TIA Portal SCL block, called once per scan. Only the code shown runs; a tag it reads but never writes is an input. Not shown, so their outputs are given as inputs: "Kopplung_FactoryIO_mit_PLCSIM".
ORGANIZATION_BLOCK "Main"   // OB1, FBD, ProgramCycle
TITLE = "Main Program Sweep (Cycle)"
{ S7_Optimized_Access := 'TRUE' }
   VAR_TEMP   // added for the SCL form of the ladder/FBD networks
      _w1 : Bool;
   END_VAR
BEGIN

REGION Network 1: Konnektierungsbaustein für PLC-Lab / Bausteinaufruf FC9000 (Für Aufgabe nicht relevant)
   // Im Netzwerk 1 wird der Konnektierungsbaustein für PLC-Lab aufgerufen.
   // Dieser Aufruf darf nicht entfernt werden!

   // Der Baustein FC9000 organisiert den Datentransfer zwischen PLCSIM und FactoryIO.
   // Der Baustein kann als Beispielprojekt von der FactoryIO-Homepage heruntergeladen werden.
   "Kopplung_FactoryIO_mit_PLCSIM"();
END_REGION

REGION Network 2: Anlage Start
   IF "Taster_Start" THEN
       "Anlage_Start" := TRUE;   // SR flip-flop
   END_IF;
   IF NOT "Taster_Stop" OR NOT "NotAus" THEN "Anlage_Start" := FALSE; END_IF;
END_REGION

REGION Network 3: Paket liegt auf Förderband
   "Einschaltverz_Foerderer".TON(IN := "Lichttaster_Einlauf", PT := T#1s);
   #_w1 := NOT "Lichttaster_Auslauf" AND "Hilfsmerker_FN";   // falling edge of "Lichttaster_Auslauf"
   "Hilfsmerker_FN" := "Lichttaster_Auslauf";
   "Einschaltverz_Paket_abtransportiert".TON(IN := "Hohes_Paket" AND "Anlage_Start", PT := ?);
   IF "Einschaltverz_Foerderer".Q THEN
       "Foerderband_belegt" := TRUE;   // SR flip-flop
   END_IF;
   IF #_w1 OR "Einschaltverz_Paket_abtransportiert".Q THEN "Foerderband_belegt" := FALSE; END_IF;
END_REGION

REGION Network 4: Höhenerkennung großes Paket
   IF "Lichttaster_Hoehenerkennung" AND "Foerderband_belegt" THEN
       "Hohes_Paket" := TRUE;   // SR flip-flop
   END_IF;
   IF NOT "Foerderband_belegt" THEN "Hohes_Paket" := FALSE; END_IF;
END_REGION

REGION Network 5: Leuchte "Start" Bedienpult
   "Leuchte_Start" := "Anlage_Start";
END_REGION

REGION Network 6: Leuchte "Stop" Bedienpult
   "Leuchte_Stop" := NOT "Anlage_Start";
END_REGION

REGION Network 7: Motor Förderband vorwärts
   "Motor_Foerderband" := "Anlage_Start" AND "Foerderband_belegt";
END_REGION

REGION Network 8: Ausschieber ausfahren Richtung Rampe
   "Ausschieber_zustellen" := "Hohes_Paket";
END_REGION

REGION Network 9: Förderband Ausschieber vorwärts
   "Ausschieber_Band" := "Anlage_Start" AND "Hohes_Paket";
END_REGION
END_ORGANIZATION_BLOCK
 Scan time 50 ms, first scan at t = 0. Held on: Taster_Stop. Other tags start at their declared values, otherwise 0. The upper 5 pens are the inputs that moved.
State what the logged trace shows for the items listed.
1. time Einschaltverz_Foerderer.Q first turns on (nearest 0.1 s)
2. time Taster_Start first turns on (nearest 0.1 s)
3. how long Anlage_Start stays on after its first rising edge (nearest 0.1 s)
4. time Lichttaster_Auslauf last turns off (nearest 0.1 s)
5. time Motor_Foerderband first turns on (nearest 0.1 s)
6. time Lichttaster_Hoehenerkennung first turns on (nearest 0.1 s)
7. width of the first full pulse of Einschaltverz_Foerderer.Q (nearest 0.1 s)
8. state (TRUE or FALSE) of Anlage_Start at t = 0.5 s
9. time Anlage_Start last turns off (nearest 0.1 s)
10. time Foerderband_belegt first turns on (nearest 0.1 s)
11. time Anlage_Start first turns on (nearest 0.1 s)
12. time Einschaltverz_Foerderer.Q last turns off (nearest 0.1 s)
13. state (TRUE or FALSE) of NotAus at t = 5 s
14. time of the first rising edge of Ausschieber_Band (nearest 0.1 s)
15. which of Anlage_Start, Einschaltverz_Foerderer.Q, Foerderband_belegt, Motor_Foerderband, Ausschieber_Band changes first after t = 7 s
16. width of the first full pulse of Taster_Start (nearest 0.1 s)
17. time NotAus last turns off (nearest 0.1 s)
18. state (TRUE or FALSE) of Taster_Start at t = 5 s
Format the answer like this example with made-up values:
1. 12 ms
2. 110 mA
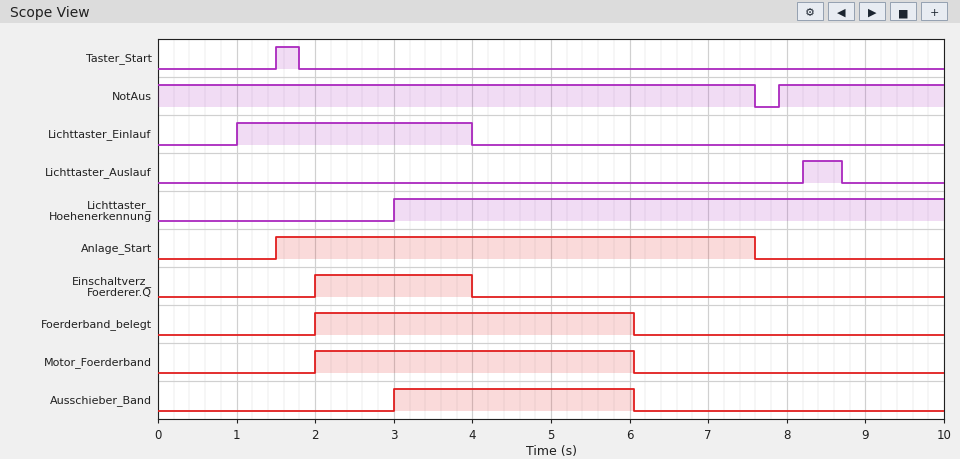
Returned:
1. 2.0 s
2. 1.5 s
3. 6.1 s
4. 8.7 s
5. 2.0 s
6. 3.0 s
7. 2.0 s
8. FALSE
9. 7.6 s
10. 2.0 s
11. 1.5 s
12. 4.0 s
13. TRUE
14. 3.0 s
15. Anlage_Start
16. 0.3 s
17. 7.6 s
18. FALSE
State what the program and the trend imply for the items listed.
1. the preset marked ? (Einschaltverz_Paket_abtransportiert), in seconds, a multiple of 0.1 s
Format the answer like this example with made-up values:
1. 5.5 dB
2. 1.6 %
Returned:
1. 3.0 s
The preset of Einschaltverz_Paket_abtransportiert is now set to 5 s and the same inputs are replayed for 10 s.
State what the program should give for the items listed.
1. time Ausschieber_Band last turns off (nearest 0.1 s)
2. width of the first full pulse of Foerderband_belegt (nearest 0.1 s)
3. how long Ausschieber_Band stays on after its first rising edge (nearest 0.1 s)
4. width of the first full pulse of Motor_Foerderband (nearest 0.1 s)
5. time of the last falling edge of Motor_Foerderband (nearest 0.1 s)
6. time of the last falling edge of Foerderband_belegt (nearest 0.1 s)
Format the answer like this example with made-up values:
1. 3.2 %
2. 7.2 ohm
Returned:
1. 7.6 s
2. 6.7 s
3. 4.6 s
4. 5.6 s
5. 7.6 s
6. 8.7 s
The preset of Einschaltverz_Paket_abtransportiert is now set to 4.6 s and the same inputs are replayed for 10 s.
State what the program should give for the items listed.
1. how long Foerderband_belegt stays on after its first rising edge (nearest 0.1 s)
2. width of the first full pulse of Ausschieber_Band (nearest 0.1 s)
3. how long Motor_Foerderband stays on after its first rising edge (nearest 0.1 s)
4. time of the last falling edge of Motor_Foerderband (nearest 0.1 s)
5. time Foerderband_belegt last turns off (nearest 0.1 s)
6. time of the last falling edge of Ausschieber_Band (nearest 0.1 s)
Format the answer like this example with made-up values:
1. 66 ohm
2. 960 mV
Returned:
1. 6.7 s
2. 4.6 s
3. 5.6 s
4. 7.6 s
5. 8.7 s
6. 7.6 s
